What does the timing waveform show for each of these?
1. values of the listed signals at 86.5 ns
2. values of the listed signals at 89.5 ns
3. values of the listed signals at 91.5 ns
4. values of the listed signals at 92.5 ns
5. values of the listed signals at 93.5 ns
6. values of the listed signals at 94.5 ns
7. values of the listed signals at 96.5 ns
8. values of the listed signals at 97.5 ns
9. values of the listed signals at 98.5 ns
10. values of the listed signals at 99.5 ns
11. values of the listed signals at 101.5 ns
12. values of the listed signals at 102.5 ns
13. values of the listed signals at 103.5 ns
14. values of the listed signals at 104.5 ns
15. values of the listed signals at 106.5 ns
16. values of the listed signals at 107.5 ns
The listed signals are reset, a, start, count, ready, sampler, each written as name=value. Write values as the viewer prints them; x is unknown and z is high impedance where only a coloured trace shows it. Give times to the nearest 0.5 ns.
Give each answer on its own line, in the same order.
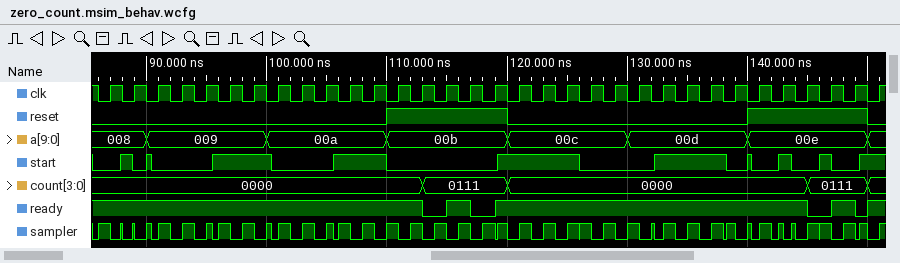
reset=0, a=008, start=0, count=0000, ready=1, sampler=1
reset=0, a=008, start=0, count=0000, ready=1, sampler=0
reset=0, a=009, start=0, count=0000, ready=1, sampler=1
reset=0, a=009, start=0, count=0000, ready=1, sampler=0
reset=0, a=009, start=0, count=0000, ready=1, sampler=1
reset=0, a=009, start=0, count=0000, ready=1, sampler=0
reset=0, a=009, start=1, count=0000, ready=1, sampler=1
reset=0, a=009, start=1, count=0000, ready=1, sampler=0
reset=0, a=009, start=1, count=0000, ready=1, sampler=1
reset=0, a=009, start=1, count=0000, ready=1, sampler=0
reset=0, a=00a, start=0, count=0000, ready=1, sampler=1
reset=0, a=00a, start=0, count=0000, ready=1, sampler=0
reset=0, a=00a, start=0, count=0000, ready=1, sampler=1
reset=0, a=00a, start=0, count=0000, ready=1, sampler=0
reset=0, a=00a, start=1, count=0000, ready=1, sampler=1
reset=0, a=00a, start=1, count=0000, ready=1, sampler=0
